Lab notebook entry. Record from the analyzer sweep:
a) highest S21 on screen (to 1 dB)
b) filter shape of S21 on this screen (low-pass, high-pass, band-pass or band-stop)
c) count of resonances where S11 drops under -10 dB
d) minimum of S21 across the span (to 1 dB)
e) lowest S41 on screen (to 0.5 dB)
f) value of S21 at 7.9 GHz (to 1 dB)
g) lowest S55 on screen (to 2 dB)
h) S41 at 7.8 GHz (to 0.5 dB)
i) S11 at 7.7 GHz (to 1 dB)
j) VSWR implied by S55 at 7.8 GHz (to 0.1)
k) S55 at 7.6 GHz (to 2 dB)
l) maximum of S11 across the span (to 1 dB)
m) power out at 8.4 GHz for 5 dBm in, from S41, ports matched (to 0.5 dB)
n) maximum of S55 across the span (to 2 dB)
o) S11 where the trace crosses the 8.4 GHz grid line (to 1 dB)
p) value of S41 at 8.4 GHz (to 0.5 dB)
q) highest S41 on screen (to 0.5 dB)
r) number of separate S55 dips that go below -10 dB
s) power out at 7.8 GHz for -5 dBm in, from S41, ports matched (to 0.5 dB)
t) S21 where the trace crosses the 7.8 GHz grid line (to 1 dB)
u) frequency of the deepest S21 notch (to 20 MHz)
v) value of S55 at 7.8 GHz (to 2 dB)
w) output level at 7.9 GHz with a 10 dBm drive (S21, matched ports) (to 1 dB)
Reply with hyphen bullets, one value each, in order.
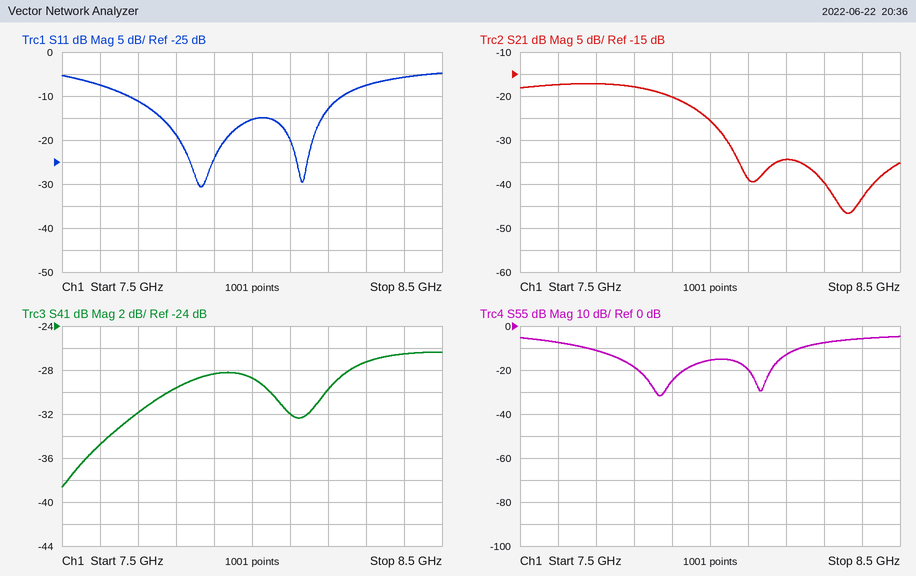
- -17 dB
- low-pass
- 2
- -47 dB
- -38.5 dB
- -20 dB
- -32 dB
- -29.5 dB
- -11 dB
- 1.3
- -8 dB
- -5 dB
- -21.5 dBm
- -4 dB
- -6 dB
- -26.5 dB
- -26.5 dB
- 2
- -34.5 dBm
- -18 dB
- 8.36 GHz
- -18 dB
- -10 dBm
